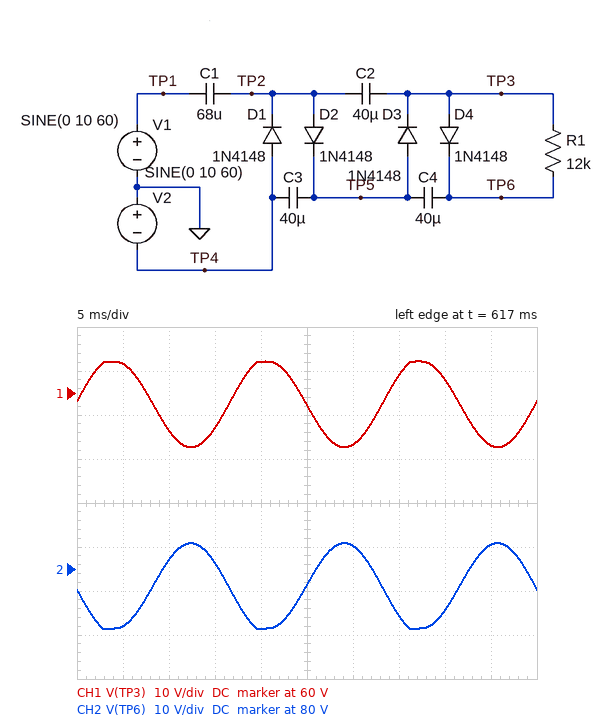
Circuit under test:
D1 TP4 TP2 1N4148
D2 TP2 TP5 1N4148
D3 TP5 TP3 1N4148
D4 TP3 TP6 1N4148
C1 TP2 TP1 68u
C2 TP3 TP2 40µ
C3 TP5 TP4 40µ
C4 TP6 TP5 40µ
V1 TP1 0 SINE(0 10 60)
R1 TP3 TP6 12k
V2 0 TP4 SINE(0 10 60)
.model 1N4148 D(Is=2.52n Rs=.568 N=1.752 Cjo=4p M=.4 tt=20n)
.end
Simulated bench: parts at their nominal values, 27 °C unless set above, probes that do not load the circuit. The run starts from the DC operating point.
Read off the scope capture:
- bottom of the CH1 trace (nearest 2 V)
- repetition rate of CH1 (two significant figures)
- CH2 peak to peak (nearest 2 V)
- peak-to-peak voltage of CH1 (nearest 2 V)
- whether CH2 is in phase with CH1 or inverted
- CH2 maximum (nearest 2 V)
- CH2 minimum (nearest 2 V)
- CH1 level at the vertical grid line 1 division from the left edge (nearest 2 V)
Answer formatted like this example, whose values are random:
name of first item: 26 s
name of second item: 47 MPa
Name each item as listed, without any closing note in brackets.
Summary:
bottom of the CH1 trace: 48 V
repetition rate of CH1: 60 Hz
CH2 peak to peak: 20 V
peak-to-peak voltage of CH1: 20 V
whether CH2 is in phase with CH1 or inverted: inverted
CH2 maximum: 86 V
CH2 minimum: 66 V
CH1 level at the vertical grid line 1 division from the left edge: 66 V
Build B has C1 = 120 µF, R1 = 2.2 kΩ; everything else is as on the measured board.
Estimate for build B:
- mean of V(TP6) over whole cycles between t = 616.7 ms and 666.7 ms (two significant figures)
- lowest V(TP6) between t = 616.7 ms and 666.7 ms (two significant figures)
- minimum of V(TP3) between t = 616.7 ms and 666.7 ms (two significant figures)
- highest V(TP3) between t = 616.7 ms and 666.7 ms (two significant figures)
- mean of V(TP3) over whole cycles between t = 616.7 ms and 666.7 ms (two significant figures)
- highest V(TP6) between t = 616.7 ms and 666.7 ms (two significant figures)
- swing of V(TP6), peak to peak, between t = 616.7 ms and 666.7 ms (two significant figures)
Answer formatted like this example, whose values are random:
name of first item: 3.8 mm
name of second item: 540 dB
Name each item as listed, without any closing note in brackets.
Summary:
mean of V(TP6) over whole cycles between t = 616.7 ms and 666.7 ms: 71 V
lowest V(TP6) between t = 616.7 ms and 666.7 ms: 62 V
minimum of V(TP3) between t = 616.7 ms and 666.7 ms: 46 V
highest V(TP3) between t = 616.7 ms and 666.7 ms: 64 V
mean of V(TP3) over whole cycles between t = 616.7 ms and 666.7 ms: 56 V
highest V(TP6) between t = 616.7 ms and 666.7 ms: 80 V
swing of V(TP6), peak to peak, between t = 616.7 ms and 666.7 ms: 18 V
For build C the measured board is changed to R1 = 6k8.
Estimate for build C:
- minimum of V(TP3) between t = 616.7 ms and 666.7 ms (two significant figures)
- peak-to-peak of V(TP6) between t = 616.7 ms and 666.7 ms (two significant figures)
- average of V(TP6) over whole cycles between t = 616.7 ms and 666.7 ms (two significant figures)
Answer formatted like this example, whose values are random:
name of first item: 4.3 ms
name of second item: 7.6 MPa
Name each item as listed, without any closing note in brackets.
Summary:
minimum of V(TP3) between t = 616.7 ms and 666.7 ms: 47 V
peak-to-peak of V(TP6) between t = 616.7 ms and 666.7 ms: 19 V
average of V(TP6) over whole cycles between t = 616.7 ms and 666.7 ms: 75 V
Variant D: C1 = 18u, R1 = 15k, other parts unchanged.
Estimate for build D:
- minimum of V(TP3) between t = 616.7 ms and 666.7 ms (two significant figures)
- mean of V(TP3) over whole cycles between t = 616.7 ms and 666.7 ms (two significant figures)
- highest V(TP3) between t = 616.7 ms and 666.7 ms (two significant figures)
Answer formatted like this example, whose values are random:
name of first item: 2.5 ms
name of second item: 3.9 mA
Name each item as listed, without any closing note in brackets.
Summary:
minimum of V(TP3) between t = 616.7 ms and 666.7 ms: 46 V
mean of V(TP3) over whole cycles between t = 616.7 ms and 666.7 ms: 56 V
highest V(TP3) between t = 616.7 ms and 666.7 ms: 66 V
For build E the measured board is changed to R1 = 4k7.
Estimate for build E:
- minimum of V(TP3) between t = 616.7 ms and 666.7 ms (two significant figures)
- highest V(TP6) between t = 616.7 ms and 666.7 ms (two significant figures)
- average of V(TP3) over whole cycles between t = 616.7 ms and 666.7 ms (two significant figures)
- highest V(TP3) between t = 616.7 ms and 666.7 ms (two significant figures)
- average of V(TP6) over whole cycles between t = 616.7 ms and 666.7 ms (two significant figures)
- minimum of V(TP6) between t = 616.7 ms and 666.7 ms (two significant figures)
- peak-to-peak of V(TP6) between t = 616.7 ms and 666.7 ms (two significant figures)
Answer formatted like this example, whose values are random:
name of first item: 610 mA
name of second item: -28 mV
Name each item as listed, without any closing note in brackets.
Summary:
minimum of V(TP3) between t = 616.7 ms and 666.7 ms: 47 V
highest V(TP6) between t = 616.7 ms and 666.7 ms: 83 V
average of V(TP3) over whole cycles between t = 616.7 ms and 666.7 ms: 57 V
highest V(TP3) between t = 616.7 ms and 666.7 ms: 66 V
average of V(TP6) over whole cycles between t = 616.7 ms and 666.7 ms: 74 V
minimum of V(TP6) between t = 616.7 ms and 666.7 ms: 65 V
peak-to-peak of V(TP6) between t = 616.7 ms and 666.7 ms: 19 V
